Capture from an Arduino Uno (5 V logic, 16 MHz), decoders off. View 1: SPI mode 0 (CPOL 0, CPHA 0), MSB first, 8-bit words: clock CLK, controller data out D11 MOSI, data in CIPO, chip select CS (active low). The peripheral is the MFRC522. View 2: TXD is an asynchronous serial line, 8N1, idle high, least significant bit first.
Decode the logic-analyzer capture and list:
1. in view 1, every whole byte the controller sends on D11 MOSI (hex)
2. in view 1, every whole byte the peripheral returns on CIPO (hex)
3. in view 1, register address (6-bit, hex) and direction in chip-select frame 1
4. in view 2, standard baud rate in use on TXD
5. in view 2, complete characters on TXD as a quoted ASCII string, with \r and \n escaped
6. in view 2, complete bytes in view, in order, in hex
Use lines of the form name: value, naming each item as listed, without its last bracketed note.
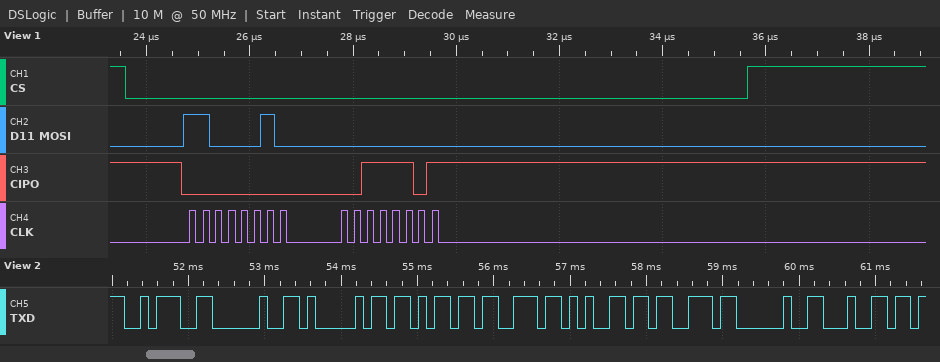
in view 1, every whole byte the controller sends on D11 MOSI: C2 00
in view 1, every whole byte the peripheral returns on CIPO: 00 3D
in view 1, register address (6-bit, hex) and direction in chip-select frame 1: 0x21 read
in view 2, standard baud rate in use on TXD: 9600 baud
in view 2, complete characters on TXD as a quoted ASCII string, with \r and \n escaped: ": Akses d"
in view 2, complete bytes in view, in order, in hex: 3A 20 41 6B 73 65 73 20 64
